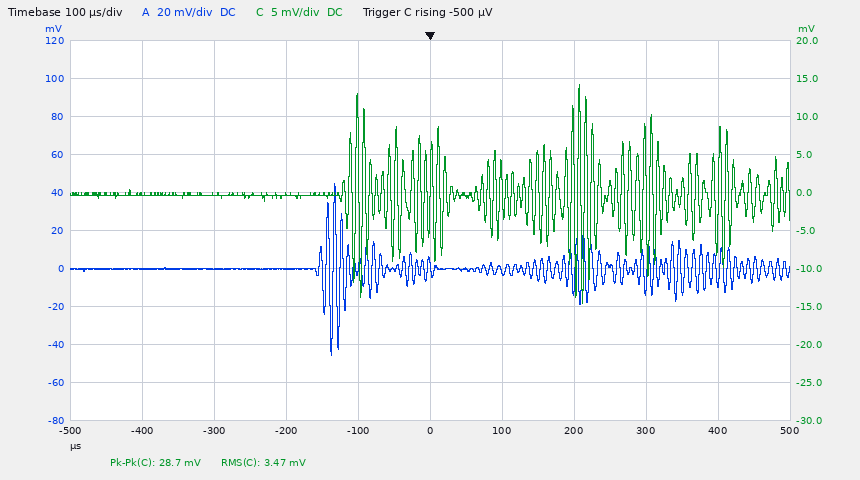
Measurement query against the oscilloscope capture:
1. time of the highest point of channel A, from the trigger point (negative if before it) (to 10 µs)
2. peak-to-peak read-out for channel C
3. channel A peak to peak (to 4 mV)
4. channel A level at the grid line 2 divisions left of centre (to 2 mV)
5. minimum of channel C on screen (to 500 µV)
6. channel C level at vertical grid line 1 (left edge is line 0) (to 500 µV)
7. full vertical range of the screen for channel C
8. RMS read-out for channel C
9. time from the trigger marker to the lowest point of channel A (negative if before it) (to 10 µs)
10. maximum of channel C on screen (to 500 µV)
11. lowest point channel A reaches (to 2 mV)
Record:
-130 µs
28.7 mV
92 mV
0 mV
-14.5 mV
0.0 mV
50 mV
3.47 mV
-140 µs
14.0 mV
-46 mV
